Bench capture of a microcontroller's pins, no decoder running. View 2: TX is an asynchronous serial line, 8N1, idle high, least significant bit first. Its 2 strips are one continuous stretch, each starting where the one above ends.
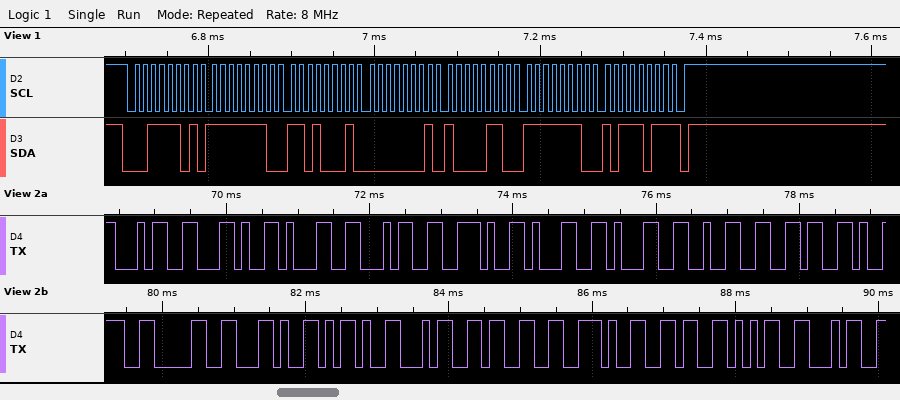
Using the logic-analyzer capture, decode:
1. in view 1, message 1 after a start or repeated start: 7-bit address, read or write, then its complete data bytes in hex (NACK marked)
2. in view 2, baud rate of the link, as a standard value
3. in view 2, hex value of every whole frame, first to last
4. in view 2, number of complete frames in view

0x1E read: FE D1 01 86 FE BB NACK
9600 baud
0x34 0x2C 0x31 0x34 0x2E 0x31 0x31 0x32 0x36 0x39 0x30 0x2C 0x2D 0x34 0x33 0x2E 0x36 0x35 0x34
19
